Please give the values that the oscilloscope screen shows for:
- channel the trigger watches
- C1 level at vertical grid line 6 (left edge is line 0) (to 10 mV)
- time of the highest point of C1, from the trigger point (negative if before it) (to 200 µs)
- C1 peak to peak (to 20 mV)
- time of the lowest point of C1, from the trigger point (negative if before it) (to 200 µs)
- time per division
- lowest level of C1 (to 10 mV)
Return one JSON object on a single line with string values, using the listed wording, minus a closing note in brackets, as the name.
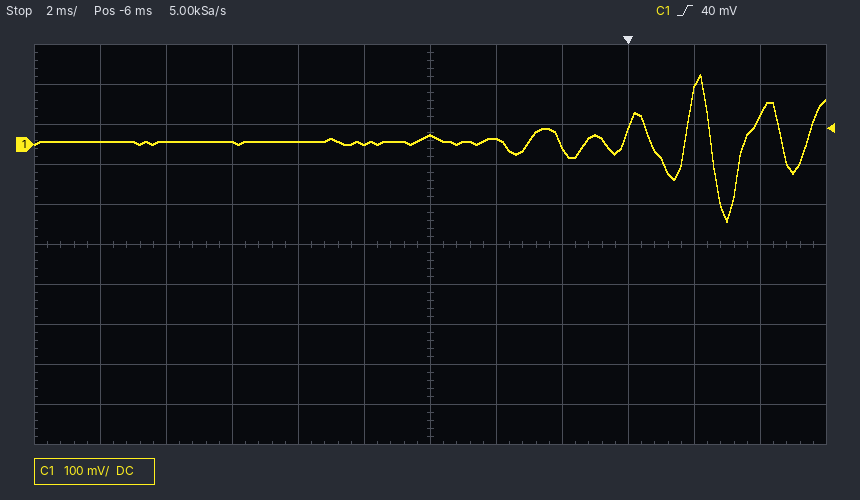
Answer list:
{"channel the trigger watches": "C1", "C1 level at vertical grid line 6 (left edge is line 0)": "20 mV", "time of the highest point of C1, from the trigger point (negative if before it)": "+2.2 ms", "C1 peak to peak": "360 mV", "time of the lowest point of C1, from the trigger point (negative if before it)": "+3.0 ms", "time per division": "2 ms", "lowest level of C1": "-190 mV"}
